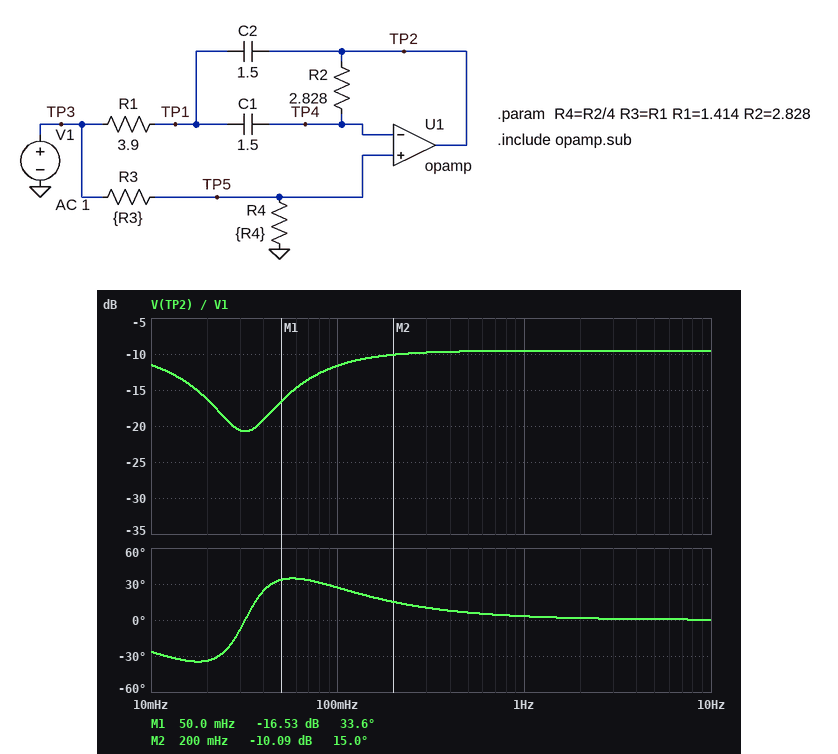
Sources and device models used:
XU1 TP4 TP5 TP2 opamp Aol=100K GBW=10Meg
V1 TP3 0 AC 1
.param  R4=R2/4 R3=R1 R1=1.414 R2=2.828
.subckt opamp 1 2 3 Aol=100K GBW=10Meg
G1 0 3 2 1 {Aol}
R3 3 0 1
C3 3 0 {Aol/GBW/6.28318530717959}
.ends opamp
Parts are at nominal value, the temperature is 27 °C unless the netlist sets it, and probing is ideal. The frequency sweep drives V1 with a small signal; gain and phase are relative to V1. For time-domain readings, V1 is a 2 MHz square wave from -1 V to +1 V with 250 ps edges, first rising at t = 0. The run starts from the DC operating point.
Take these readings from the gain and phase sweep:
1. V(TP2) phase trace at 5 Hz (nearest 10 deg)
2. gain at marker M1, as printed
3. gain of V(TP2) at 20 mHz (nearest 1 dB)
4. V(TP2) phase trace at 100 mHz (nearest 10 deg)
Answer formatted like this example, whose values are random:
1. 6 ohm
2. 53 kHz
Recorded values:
1. 0 deg
2. -16.53 dB
3. -16 dB
4. 30 deg
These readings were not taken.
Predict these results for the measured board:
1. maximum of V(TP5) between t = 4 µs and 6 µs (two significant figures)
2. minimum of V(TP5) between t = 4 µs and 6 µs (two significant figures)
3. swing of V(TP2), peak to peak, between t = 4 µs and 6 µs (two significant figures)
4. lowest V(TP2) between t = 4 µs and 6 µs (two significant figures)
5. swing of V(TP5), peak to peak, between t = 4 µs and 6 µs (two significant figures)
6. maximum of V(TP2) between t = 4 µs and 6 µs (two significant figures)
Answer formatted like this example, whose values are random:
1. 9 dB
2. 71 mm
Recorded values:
1. 330 mV
2. -330 mV
3. 670 mV
4. -330 mV
5. 670 mV
6. 330 mV
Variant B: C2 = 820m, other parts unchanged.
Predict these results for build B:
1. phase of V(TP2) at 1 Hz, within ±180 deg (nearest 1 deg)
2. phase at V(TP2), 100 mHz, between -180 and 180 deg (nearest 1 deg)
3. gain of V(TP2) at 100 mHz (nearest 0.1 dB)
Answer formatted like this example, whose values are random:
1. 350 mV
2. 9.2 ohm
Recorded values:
1. 6 deg
2. 48 deg
3. -13.8 dB
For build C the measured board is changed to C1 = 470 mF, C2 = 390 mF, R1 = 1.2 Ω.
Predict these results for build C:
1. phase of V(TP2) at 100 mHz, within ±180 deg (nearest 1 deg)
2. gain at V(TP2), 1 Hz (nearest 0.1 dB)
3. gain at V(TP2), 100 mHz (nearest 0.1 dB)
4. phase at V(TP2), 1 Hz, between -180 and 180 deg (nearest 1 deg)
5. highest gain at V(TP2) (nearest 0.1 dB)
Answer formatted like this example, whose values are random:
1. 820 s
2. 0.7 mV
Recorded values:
1. -94 deg
2. -9.1 dB
3. -7.4 dB
4. 39 deg
5. -5.6 dB
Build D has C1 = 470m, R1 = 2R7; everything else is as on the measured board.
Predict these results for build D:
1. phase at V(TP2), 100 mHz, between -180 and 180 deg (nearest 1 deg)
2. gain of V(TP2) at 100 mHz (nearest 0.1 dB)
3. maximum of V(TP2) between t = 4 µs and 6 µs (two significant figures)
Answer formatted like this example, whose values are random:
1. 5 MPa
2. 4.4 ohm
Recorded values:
1. 15 deg
2. -14.4 dB
3. 330 mV
